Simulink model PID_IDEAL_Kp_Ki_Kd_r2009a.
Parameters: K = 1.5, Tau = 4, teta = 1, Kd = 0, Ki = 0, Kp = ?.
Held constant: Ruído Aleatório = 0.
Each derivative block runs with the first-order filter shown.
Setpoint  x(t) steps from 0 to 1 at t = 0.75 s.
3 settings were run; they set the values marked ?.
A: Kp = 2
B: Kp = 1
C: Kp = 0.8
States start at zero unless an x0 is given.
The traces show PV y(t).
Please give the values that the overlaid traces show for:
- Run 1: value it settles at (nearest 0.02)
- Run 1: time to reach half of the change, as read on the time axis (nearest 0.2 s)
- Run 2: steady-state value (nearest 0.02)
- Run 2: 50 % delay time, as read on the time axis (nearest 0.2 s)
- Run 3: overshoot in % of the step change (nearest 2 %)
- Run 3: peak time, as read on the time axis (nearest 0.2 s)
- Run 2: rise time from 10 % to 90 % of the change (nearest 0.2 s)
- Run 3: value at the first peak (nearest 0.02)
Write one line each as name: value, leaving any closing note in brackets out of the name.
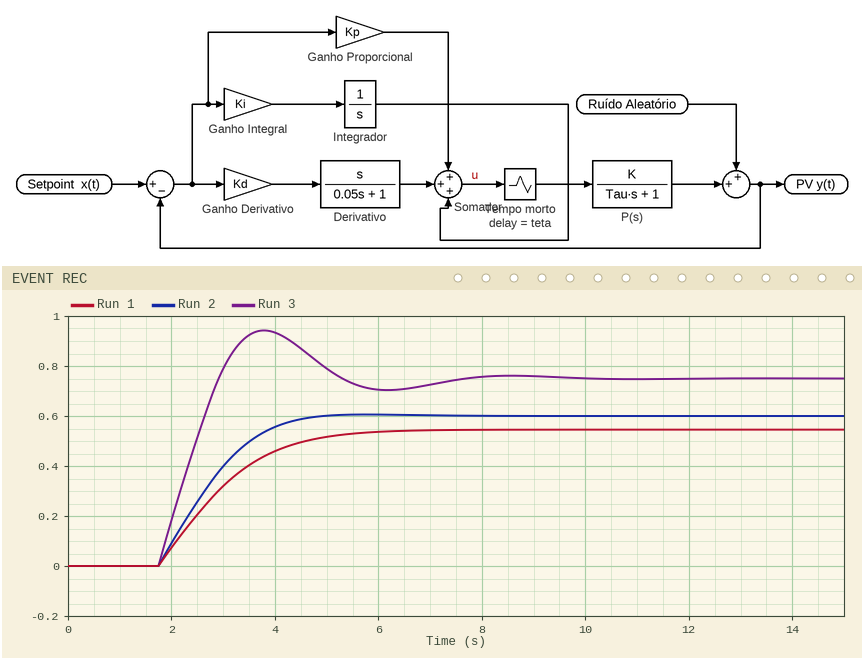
Run 1: value it settles at: 0.54
Run 1: time to reach half of the change, as read on the time axis: 2.8 s
Run 2: steady-state value: 0.60
Run 2: 50 % delay time, as read on the time axis: 2.6 s
Run 3: overshoot in % of the step change: 26 %
Run 3: peak time, as read on the time axis: 3.8 s
Run 2: rise time from 10 % to 90 % of the change: 2.0 s
Run 3: value at the first peak: 0.94
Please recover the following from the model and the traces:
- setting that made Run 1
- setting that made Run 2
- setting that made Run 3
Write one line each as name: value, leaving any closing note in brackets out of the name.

setting that made Run 1: C
setting that made Run 2: B
setting that made Run 3: A
